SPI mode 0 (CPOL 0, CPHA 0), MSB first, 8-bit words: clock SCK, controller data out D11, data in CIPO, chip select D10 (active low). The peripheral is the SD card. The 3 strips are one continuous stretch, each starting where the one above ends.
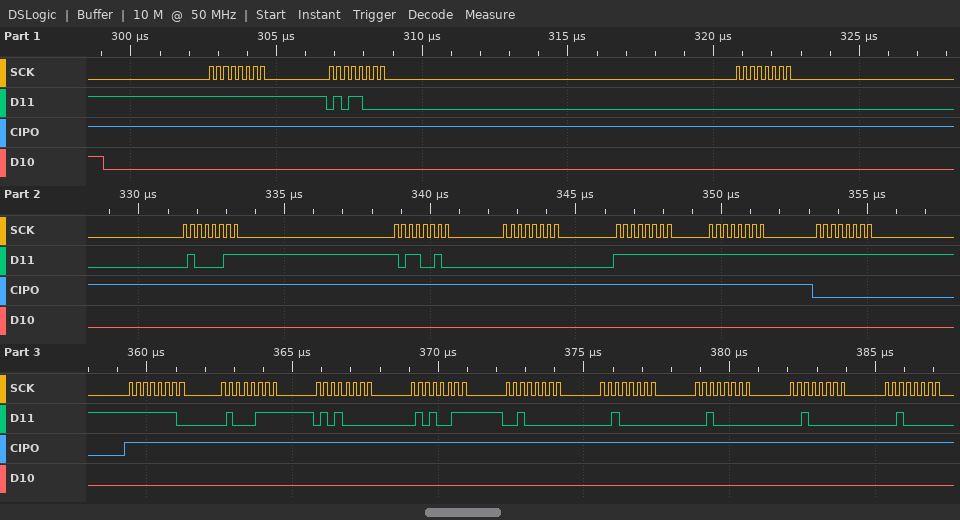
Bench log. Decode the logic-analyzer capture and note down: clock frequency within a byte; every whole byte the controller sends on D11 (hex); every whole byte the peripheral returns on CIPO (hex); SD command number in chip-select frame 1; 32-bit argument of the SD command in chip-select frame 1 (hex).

4 MHz
FF 58 00 43 B2 00 FF FF FF FE 47 50 53 20 20 20 20 20
FF FF FF FF FF FF FF FF 00 FF FF FF FF FF FF FF FF FF
CMD24
0x0043B200
